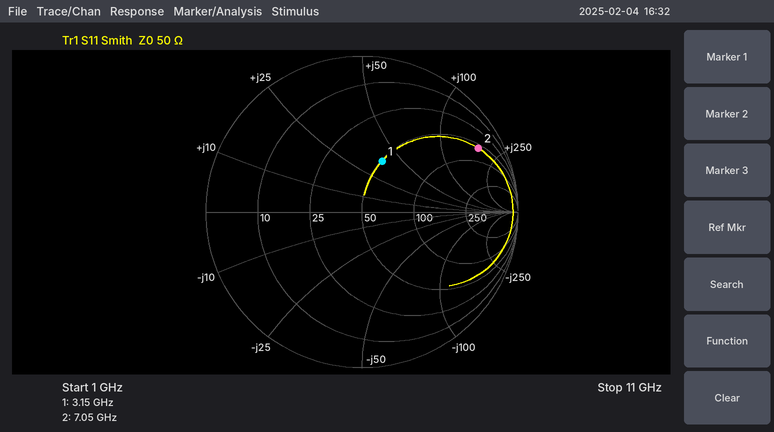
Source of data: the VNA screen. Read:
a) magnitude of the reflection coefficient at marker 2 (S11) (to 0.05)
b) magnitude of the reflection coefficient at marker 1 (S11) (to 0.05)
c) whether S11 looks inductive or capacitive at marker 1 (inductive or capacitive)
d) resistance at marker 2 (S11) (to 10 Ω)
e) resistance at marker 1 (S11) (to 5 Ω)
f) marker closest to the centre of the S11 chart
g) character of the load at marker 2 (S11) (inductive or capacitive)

0.85
0.35
inductive
60 Ω
50 Ω
marker 1
inductive
